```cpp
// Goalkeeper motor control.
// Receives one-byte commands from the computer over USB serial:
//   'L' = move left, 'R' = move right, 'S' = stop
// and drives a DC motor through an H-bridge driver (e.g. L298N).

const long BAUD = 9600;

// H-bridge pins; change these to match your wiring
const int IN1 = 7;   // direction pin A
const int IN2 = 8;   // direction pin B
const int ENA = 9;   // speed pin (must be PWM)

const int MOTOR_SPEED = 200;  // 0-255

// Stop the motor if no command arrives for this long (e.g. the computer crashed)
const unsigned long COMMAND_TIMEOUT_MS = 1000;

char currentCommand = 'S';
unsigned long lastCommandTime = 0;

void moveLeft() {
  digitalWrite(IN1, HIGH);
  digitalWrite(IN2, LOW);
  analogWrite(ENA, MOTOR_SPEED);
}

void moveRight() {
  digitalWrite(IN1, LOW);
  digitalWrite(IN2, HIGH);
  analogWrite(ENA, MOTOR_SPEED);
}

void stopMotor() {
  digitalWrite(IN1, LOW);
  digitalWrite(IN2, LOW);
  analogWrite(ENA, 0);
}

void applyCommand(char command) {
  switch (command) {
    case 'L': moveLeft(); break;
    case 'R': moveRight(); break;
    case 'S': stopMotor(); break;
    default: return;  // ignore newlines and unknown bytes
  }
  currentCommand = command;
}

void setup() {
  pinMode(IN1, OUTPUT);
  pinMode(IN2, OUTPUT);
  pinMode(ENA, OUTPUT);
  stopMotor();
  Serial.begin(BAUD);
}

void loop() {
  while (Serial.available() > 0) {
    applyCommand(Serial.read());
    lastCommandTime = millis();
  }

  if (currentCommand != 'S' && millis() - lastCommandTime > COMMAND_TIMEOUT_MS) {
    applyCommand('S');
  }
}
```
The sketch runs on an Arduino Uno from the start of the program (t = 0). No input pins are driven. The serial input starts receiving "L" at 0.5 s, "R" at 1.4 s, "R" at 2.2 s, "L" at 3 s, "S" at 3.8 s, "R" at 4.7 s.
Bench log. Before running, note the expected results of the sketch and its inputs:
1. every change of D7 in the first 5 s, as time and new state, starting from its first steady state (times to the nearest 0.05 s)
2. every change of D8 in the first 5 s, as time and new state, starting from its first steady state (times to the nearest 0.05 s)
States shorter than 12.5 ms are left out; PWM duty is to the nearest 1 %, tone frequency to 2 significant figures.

0 s low; 0.5 s high; 1.4 s low; 3 s high; 3.8 s low
0 s low; 1.4 s high; 3 s low; 4.7 s high
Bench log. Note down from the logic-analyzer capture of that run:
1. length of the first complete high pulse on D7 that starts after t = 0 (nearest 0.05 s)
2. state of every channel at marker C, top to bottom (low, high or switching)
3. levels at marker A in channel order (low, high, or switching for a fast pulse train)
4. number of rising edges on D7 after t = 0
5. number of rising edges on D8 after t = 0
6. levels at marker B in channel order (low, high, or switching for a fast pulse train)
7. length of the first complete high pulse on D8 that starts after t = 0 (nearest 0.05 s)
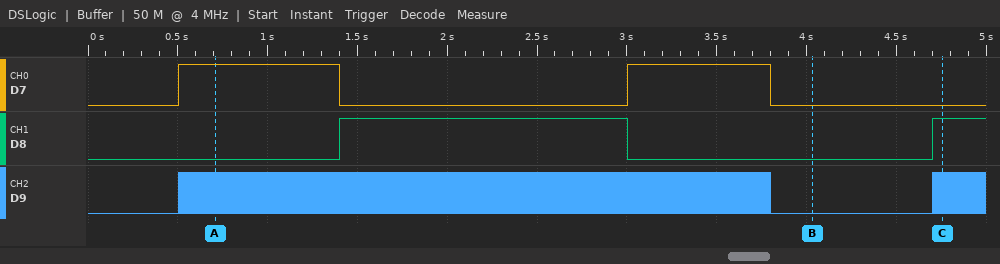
0.90 s
D7 low, D8 high, D9 switching
D7 high, D8 low, D9 switching
2
2
D7 low, D8 low, D9 low
1.60 s
